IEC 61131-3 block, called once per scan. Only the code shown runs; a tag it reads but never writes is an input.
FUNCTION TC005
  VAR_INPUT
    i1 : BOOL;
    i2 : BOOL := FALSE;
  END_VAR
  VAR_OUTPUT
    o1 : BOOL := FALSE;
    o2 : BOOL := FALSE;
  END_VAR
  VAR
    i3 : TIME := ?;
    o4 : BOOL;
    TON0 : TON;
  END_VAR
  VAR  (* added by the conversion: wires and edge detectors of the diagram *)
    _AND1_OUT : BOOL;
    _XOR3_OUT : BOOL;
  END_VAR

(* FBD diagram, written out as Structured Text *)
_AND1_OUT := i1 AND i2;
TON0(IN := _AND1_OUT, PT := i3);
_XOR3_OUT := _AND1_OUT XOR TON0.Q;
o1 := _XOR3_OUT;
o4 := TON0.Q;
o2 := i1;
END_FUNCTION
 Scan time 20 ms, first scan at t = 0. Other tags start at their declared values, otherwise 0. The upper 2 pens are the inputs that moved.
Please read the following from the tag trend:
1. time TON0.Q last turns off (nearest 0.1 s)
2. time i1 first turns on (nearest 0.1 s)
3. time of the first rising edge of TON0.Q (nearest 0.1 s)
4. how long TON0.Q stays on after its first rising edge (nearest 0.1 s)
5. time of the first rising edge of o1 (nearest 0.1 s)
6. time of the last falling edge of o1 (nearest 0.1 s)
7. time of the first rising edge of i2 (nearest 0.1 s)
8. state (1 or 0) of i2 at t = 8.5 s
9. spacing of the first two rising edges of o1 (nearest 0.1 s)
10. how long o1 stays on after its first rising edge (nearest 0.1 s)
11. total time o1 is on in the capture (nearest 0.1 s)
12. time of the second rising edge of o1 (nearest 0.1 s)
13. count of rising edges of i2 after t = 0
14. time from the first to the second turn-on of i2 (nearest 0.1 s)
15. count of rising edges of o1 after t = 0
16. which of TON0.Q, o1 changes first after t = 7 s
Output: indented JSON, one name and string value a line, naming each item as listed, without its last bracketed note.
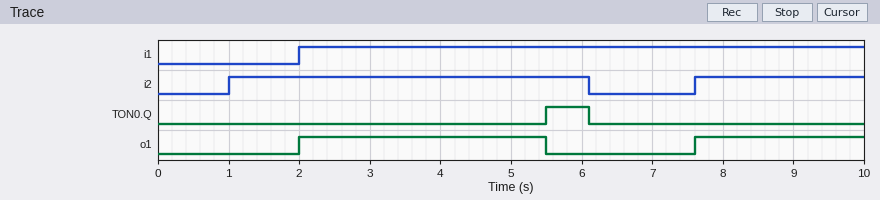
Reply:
{
  "time TON0.Q last turns off": "6.1 s",
  "time i1 first turns on": "2.0 s",
  "time of the first rising edge of TON0.Q": "5.5 s",
  "how long TON0.Q stays on after its first rising edge": "0.6 s",
  "time of the first rising edge of o1": "2.0 s",
  "time of the last falling edge of o1": "5.5 s",
  "time of the first rising edge of i2": "1.0 s",
  "state (1 or 0) of i2 at t = 8.5 s": "1",
  "spacing of the first two rising edges of o1": "5.6 s",
  "how long o1 stays on after its first rising edge": "3.5 s",
  "total time o1 is on in the capture": "5.9 s",
  "time of the second rising edge of o1": "7.6 s",
  "count of rising edges of i2 after t = 0": "2",
  "time from the first to the second turn-on of i2": "6.6 s",
  "count of rising edges of o1 after t = 0": "2",
  "which of TON0.Q, o1 changes first after t = 7 s": "o1"
}
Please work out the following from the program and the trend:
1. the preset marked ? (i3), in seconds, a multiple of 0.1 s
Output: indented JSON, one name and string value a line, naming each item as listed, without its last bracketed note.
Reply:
{
  "the preset marked ? (i3), in seconds, a multiple of 0.1 s": "3.5 s"
}
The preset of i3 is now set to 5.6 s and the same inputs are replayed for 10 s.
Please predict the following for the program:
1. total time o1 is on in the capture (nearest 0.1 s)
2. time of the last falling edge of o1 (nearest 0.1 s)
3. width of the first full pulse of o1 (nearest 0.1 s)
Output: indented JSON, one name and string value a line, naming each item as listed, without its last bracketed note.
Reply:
{
  "total time o1 is on in the capture": "6.5 s",
  "time of the last falling edge of o1": "6.1 s",
  "width of the first full pulse of o1": "4.1 s"
}
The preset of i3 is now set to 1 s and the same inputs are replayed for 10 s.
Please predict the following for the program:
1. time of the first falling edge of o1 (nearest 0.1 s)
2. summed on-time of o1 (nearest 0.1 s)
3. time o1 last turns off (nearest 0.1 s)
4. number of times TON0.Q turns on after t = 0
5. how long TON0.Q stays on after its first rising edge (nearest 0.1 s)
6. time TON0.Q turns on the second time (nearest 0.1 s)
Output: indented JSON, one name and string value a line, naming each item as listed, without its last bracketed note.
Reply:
{
  "time of the first falling edge of o1": "3.0 s",
  "summed on-time of o1": "2.0 s",
  "time o1 last turns off": "8.6 s",
  "number of times TON0.Q turns on after t = 0": "2",
  "how long TON0.Q stays on after its first rising edge": "3.1 s",
  "time TON0.Q turns on the second time": "8.6 s"
}
